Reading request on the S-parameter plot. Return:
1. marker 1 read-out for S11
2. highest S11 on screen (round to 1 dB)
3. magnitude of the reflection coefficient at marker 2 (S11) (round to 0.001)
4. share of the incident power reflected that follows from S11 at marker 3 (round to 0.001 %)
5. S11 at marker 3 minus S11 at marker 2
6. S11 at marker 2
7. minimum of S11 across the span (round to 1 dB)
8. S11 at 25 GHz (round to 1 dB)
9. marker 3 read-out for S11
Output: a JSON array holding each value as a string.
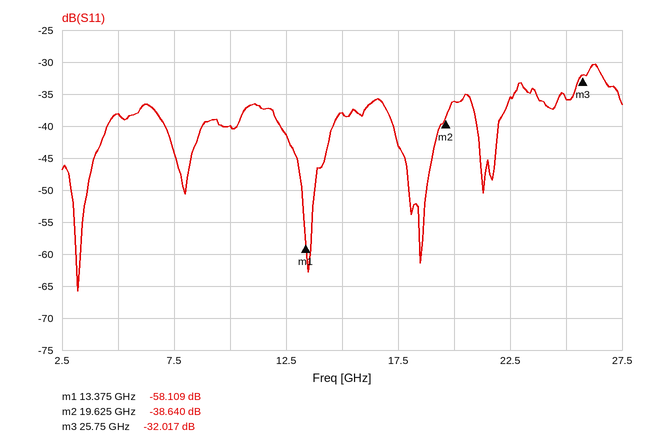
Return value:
["-58.109 dB", "-30 dB", "0.012", "0.063 %", "6.623 dB", "-38.640 dB", "-66 dB", "-36 dB", "-32.017 dB"]
